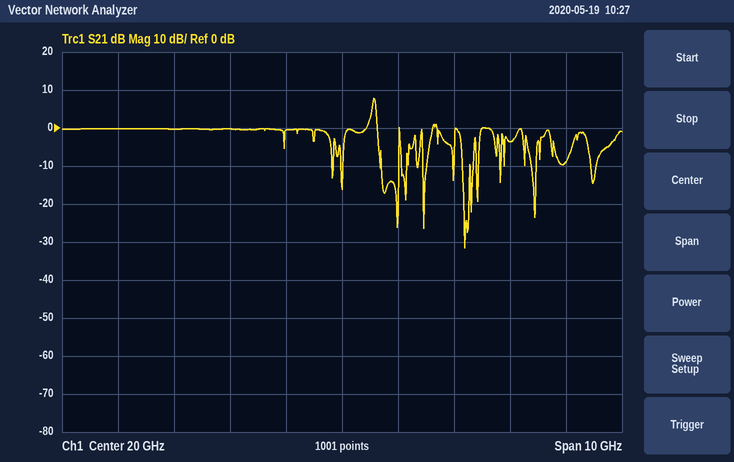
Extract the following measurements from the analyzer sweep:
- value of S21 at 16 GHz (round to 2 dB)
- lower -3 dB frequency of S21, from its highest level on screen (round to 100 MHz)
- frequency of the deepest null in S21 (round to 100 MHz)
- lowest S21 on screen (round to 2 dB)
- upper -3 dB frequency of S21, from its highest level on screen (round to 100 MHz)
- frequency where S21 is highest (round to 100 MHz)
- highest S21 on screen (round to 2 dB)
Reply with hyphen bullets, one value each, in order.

- 0 dB
- 20.5 GHz
- 22.2 GHz
- -32 dB
- 20.6 GHz
- 20.6 GHz
- 8 dB
